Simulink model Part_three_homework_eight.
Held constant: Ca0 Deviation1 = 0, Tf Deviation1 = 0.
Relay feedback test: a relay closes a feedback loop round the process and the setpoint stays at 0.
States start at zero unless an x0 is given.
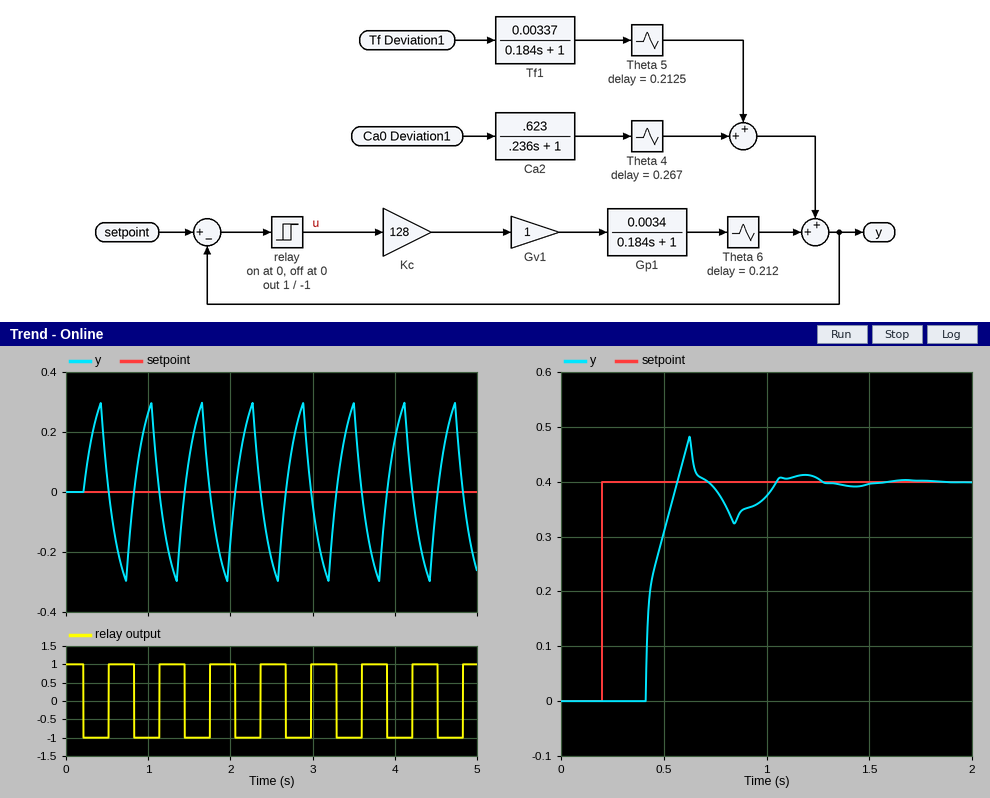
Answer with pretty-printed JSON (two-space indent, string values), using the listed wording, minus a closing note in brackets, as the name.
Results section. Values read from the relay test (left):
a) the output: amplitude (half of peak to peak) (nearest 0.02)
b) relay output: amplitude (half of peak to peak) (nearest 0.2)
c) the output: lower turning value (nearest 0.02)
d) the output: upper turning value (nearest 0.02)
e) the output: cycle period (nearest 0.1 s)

{
  "the output: amplitude (half of peak to peak)": "0.30",
  "relay output: amplitude (half of peak to peak)": "1.0",
  "the output: lower turning value": "-0.30",
  "the output: upper turning value": "0.30",
  "the output: cycle period": "0.6 s"
}
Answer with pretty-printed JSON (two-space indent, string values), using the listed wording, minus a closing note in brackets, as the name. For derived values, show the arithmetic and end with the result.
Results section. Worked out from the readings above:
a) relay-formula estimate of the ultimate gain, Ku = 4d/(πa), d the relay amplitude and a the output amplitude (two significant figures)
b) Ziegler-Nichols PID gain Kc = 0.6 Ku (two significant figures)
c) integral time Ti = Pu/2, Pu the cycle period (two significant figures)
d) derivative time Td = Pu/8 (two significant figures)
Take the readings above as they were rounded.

{
  "relay-formula estimate of the ultimate gain, Ku = 4d/(πa), d the relay amplitude and a the output amplitude": "4 × 1 / (π × 0.3) = 4.2",
  "Ziegler-Nichols PID gain Kc = 0.6 Ku": "0.6 × 4.2 = 2.5",
  "integral time Ti = Pu/2, Pu the cycle period": "0.6 / 2 = 0.30 s",
  "derivative time Td = Pu/8": "0.6 / 8 = 0.075 s"
}
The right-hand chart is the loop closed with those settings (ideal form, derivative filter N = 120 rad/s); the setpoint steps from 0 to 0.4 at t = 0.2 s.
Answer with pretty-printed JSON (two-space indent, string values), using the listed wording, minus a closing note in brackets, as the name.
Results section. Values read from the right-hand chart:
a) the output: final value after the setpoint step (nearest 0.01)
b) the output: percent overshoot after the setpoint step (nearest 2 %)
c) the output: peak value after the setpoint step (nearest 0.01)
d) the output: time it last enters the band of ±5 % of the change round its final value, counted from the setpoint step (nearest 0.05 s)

{
  "the output: final value after the setpoint step": "0.40",
  "the output: percent overshoot after the setpoint step": "20 %",
  "the output: peak value after the setpoint step": "0.48",
  "the output: time it last enters the band of ±5 % of the change round its final value, counted from the setpoint step": "0.80 s"
}
